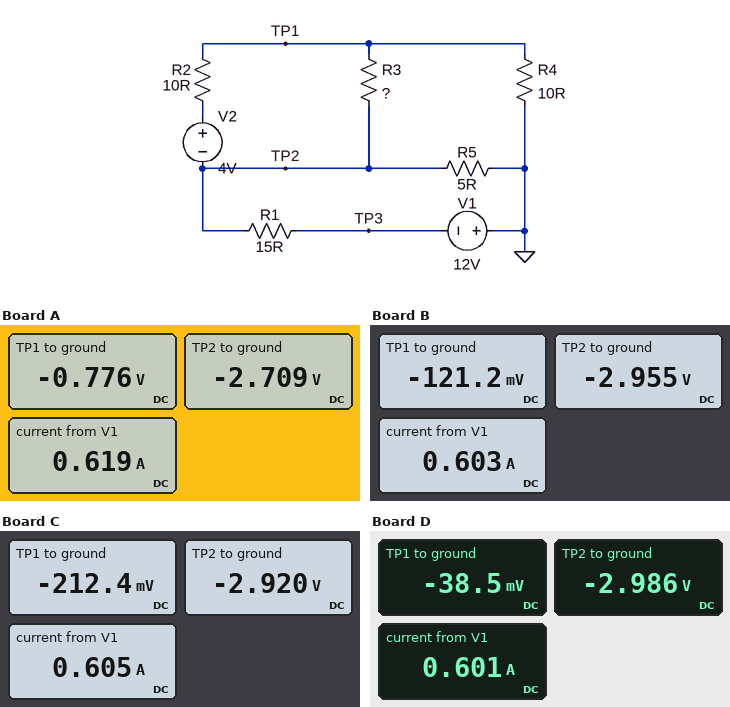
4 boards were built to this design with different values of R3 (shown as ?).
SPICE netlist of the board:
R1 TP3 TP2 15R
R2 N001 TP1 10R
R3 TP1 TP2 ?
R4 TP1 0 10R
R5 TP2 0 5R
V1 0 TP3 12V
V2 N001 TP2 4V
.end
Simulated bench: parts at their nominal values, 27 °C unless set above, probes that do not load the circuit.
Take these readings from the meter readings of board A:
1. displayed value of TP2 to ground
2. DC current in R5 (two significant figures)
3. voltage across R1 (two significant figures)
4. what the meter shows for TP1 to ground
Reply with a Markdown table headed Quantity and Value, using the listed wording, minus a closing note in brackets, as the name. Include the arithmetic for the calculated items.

| Quantity | Value |
|---|---|
| displayed value of TP2 to ground | -2.709 V |
| DC current in R5 | (0 V - (-2.709 V)) / 5 Ω = 540 mA |
| voltage across R1 | -2.709 V - (-12 V) = 9.3 V |
| what the meter shows for TP1 to ground | -0.776 V |
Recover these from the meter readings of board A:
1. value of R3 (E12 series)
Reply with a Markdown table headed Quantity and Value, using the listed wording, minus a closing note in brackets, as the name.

| Quantity | Value |
|---|---|
| value of R3 | 6.8 Ω |
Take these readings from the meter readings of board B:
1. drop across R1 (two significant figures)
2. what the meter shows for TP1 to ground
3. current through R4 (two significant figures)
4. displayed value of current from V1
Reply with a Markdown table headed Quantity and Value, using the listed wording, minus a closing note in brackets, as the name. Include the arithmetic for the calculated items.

| Quantity | Value |
|---|---|
| drop across R1 | -2.955 V - (-12 V) = 9.0 V |
| what the meter shows for TP1 to ground | -121.2 mV |
| current through R4 | (0 V - (-121.2 mV)) / 10 Ω = 12 mA |
| displayed value of current from V1 | 0.603 A |
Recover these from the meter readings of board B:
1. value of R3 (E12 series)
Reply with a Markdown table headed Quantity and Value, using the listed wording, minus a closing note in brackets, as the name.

| Quantity | Value |
|---|---|
| value of R3 | 22 Ω |
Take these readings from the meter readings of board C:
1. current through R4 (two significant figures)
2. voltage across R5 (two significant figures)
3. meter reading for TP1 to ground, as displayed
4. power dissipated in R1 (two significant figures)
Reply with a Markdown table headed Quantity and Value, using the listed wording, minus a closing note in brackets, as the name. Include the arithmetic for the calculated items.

| Quantity | Value |
|---|---|
| current through R4 | (0 V - (-212.4 mV)) / 10 Ω = 21 mA |
| voltage across R5 | 0 V - (-2.92 V) = 2.9 V |
| meter reading for TP1 to ground, as displayed | -212.4 mV |
| power dissipated in R1 | (-2.92 V - (-12 V))^2 / 15 Ω = 5.5 W |
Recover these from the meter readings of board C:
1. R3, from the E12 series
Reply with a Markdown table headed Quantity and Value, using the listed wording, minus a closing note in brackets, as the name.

| Quantity | Value |
|---|---|
| R3, from the E12 series | 18 Ω |
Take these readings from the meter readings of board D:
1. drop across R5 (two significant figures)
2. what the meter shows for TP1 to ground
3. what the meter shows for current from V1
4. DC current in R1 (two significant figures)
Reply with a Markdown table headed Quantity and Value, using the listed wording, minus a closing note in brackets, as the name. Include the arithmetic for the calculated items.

| Quantity | Value |
|---|---|
| drop across R5 | 0 V - (-2.986 V) = 3.0 V |
| what the meter shows for TP1 to ground | -38.5 mV |
| what the meter shows for current from V1 | 0.601 A |
| DC current in R1 | (-2.986 V - (-12 V)) / 15 Ω = 600 mA |
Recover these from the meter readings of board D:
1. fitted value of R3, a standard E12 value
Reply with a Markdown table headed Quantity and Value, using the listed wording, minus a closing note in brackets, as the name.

| Quantity | Value |
|---|---|
| fitted value of R3, a standard E12 value | 27 Ω |
